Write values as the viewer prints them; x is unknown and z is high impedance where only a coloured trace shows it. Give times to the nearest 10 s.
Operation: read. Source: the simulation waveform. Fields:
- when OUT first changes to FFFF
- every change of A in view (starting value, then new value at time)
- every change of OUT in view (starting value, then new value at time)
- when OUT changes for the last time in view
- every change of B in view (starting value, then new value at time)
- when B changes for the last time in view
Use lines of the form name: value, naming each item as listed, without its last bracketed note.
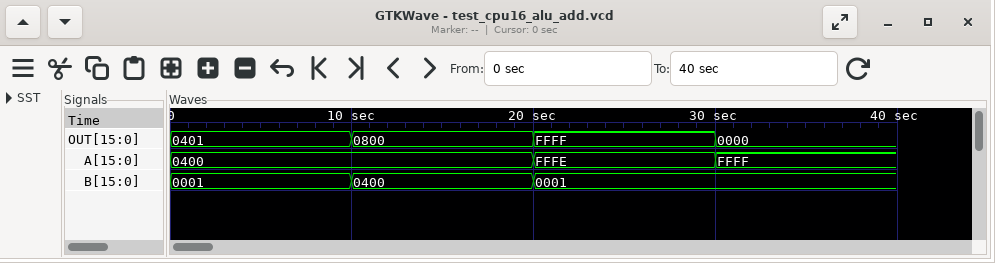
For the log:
when OUT first changes to FFFF: 20 s
every change of A in view: 0400, FFFE at 20 s, FFFF at 30 s
every change of OUT in view: 0401, 0800 at 10 s, FFFF at 20 s, 0000 at 30 s
when OUT changes for the last time in view: 30 s
every change of B in view: 0001, 0400 at 10 s, 0001 at 20 s
when B changes for the last time in view: 20 s
